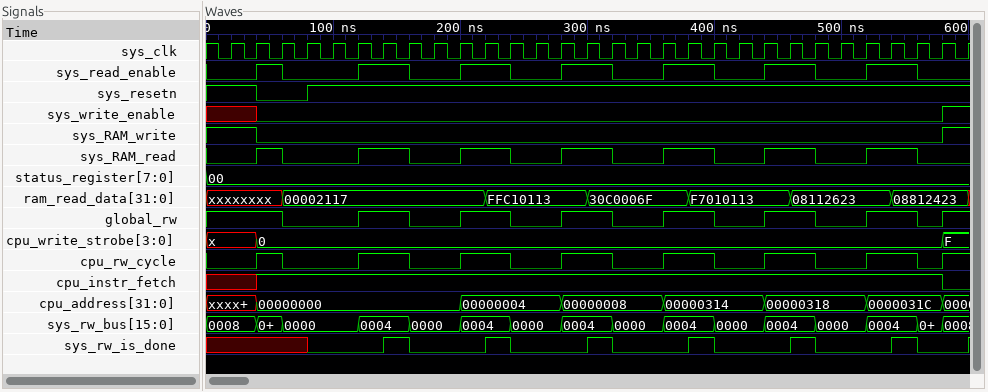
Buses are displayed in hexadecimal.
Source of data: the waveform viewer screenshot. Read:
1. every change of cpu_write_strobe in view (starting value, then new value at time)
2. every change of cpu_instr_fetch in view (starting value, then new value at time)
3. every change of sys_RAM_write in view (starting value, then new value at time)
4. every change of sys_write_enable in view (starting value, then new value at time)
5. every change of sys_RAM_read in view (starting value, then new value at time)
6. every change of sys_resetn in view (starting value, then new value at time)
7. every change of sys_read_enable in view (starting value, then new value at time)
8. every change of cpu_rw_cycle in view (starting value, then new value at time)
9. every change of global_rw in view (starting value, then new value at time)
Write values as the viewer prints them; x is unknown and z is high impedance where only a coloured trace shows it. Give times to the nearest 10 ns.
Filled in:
x, 0 at 40 ns, F at 580 ns
x, 1 at 40 ns, 0 at 580 ns
1, 0 at 40 ns, 1 at 580 ns
x, 0 at 40 ns, 1 at 580 ns
0, 1 at 40 ns, 0 at 60 ns, 1 at 120 ns, 0 at 160 ns, 1 at 200 ns, 0 at 240 ns, 1 at 280 ns, 0 at 320 ns, 1 at 360 ns, 0 at 400 ns, 1 at 440 ns, 0 at 480 ns, 1 at 520 ns, 0 at 560 ns
1, 0 at 40 ns, 1 at 80 ns
0, 1 at 40 ns, 0 at 60 ns, 1 at 120 ns, 0 at 160 ns, 1 at 200 ns, 0 at 240 ns, 1 at 280 ns, 0 at 320 ns, 1 at 360 ns, 0 at 400 ns, 1 at 440 ns, 0 at 480 ns, 1 at 520 ns, 0 at 560 ns
0, 1 at 40 ns, 0 at 60 ns, 1 at 120 ns, 0 at 160 ns, 1 at 200 ns, 0 at 240 ns, 1 at 280 ns, 0 at 320 ns, 1 at 360 ns, 0 at 400 ns, 1 at 440 ns, 0 at 480 ns, 1 at 520 ns, 0 at 560 ns, 1 at 580 ns
1, 0 at 60 ns, 1 at 120 ns, 0 at 160 ns, 1 at 200 ns, 0 at 240 ns, 1 at 280 ns, 0 at 320 ns, 1 at 360 ns, 0 at 400 ns, 1 at 440 ns, 0 at 480 ns, 1 at 520 ns, 0 at 560 ns, 1 at 580 ns
